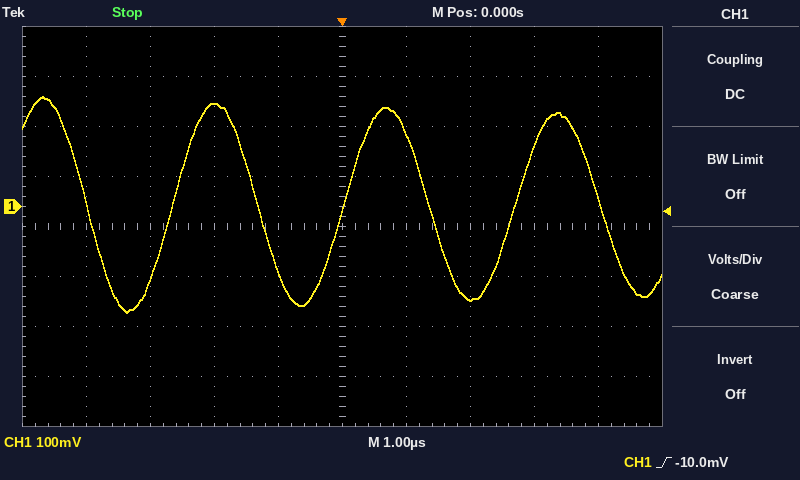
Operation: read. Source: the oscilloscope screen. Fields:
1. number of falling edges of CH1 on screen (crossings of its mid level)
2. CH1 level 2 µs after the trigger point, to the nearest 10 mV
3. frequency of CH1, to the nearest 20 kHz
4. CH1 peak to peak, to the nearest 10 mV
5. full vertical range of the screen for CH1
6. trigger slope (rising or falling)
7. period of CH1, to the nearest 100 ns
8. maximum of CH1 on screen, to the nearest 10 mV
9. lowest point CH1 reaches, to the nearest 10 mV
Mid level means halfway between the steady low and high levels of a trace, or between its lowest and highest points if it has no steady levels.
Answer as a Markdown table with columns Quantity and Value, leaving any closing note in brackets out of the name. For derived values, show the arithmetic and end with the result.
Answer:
| Quantity | Value |
|---|---|
| number of falling edges of CH1 on screen | 4 |
| CH1 level 2 µs after the trigger point, to the nearest 10 mV | -190 mV |
| frequency of CH1, to the nearest 20 kHz | 1 / 2.7 µs ≈ 370 kHz, so 380 kHz to the nearest 20 kHz |
| CH1 peak to peak, to the nearest 10 mV | 220 mV − (-210 mV) = 430 mV |
| full vertical range of the screen for CH1 | 800 mV |
| trigger slope | rising |
| period of CH1, to the nearest 100 ns | 2.7 µs |
| maximum of CH1 on screen, to the nearest 10 mV | 220 mV |
| lowest point CH1 reaches, to the nearest 10 mV | -210 mV |
